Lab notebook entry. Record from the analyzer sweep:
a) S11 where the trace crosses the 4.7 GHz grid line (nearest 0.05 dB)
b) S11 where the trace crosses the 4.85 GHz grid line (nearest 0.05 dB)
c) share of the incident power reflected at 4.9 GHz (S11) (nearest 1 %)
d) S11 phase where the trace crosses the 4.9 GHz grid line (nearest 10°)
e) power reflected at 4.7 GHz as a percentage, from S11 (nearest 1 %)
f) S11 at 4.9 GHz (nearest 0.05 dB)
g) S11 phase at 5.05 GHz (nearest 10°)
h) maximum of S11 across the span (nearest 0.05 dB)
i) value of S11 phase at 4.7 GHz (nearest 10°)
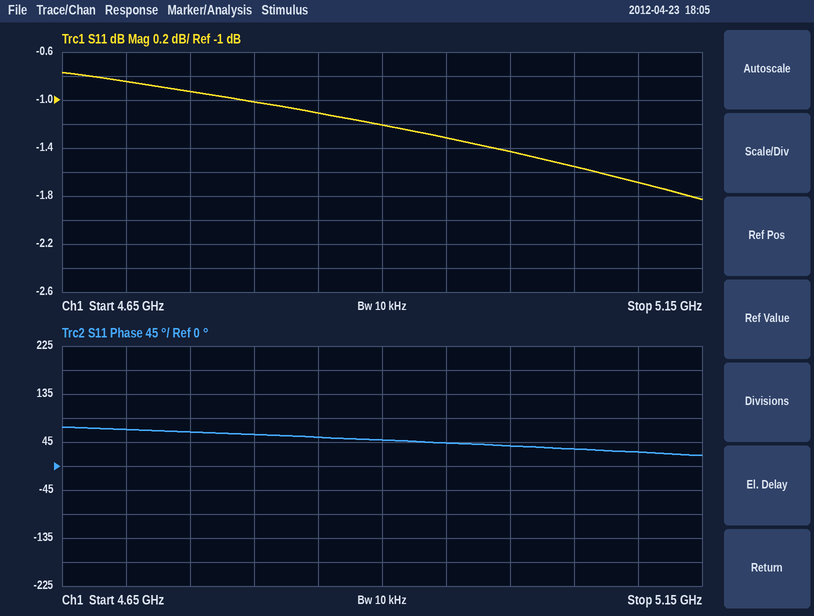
-0.85 dB
-1.10 dB
76 %
50°
82 %
-1.20 dB
30°
-0.75 dB
70°
